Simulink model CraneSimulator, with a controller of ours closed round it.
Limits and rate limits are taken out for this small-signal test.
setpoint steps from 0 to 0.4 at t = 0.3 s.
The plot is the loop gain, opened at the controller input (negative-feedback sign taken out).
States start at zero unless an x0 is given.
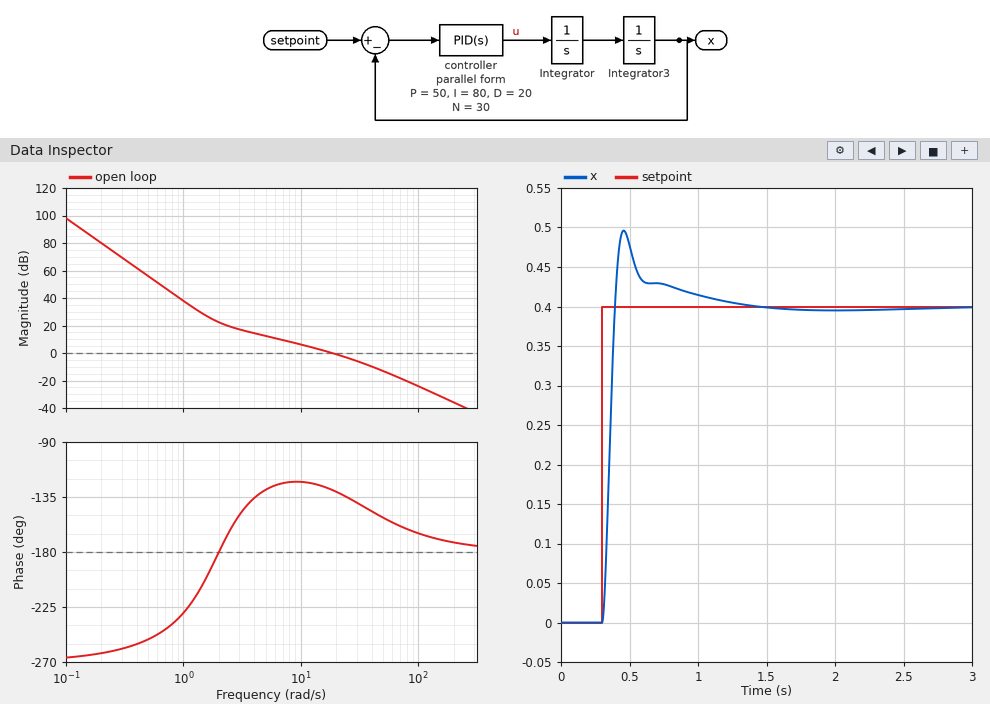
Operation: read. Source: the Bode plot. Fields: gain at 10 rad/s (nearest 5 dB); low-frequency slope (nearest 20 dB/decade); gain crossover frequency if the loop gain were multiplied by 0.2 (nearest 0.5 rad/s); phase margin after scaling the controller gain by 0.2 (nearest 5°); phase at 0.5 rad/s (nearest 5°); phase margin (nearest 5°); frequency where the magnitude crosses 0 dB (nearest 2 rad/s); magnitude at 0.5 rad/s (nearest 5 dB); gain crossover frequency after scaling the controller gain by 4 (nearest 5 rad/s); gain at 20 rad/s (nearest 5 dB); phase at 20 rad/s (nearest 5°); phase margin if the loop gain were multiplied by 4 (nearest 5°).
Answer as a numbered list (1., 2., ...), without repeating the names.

1. 5 dB
2. -60 dB/decade
3. 4.0 rad/s
4. 45°
5. -250°
6. 50°
7. 18 rad/s
8. 55 dB
9. 45 rad/s
10. 0 dB
11. -130°
12. 30°
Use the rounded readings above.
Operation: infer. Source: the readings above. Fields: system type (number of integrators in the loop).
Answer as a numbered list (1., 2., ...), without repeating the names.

1. 3
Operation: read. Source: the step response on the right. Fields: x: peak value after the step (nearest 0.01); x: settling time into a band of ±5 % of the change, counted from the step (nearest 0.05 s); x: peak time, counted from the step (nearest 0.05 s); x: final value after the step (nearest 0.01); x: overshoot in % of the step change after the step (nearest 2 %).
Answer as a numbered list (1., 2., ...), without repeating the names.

1. 0.50
2. 0.60 s
3. 0.15 s
4. 0.40
5. 24 %
